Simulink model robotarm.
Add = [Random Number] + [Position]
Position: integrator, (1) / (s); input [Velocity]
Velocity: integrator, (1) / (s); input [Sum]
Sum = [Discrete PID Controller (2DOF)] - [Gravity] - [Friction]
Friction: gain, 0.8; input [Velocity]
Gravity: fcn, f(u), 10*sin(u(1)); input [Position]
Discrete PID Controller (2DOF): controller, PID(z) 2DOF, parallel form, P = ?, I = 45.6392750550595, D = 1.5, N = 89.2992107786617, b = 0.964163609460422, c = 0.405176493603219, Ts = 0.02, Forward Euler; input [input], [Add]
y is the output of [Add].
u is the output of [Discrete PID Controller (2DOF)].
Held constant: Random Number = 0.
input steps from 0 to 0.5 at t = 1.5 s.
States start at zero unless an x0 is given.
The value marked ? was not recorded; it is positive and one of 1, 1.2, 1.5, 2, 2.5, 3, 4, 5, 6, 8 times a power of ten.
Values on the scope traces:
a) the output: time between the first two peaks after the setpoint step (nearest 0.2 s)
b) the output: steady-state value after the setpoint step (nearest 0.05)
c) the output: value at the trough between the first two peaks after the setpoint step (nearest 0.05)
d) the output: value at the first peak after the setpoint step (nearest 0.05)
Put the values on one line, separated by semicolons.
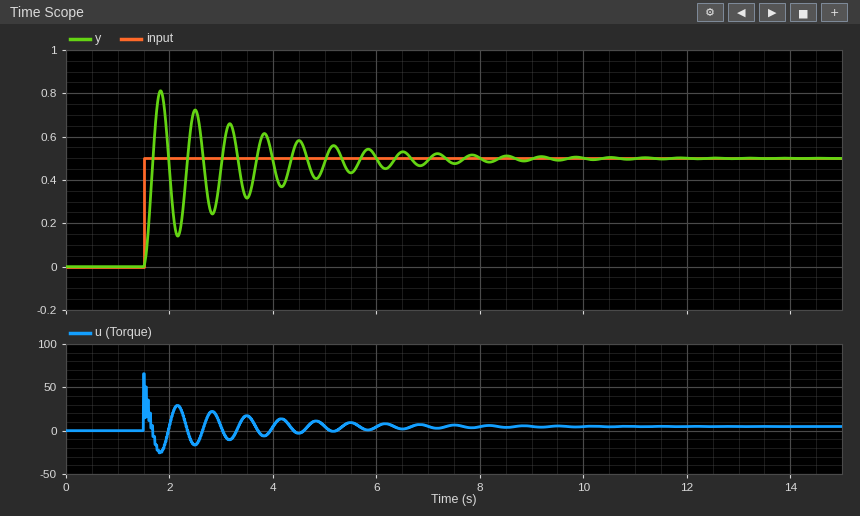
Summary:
0.6 s; 0.50; 0.15; 0.80
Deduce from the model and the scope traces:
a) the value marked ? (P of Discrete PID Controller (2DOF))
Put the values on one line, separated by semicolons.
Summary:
80
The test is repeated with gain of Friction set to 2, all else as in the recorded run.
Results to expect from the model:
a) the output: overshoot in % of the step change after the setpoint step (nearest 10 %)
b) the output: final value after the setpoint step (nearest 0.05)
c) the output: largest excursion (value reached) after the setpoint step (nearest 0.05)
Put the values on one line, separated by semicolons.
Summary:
50 %; 0.50; 0.75
